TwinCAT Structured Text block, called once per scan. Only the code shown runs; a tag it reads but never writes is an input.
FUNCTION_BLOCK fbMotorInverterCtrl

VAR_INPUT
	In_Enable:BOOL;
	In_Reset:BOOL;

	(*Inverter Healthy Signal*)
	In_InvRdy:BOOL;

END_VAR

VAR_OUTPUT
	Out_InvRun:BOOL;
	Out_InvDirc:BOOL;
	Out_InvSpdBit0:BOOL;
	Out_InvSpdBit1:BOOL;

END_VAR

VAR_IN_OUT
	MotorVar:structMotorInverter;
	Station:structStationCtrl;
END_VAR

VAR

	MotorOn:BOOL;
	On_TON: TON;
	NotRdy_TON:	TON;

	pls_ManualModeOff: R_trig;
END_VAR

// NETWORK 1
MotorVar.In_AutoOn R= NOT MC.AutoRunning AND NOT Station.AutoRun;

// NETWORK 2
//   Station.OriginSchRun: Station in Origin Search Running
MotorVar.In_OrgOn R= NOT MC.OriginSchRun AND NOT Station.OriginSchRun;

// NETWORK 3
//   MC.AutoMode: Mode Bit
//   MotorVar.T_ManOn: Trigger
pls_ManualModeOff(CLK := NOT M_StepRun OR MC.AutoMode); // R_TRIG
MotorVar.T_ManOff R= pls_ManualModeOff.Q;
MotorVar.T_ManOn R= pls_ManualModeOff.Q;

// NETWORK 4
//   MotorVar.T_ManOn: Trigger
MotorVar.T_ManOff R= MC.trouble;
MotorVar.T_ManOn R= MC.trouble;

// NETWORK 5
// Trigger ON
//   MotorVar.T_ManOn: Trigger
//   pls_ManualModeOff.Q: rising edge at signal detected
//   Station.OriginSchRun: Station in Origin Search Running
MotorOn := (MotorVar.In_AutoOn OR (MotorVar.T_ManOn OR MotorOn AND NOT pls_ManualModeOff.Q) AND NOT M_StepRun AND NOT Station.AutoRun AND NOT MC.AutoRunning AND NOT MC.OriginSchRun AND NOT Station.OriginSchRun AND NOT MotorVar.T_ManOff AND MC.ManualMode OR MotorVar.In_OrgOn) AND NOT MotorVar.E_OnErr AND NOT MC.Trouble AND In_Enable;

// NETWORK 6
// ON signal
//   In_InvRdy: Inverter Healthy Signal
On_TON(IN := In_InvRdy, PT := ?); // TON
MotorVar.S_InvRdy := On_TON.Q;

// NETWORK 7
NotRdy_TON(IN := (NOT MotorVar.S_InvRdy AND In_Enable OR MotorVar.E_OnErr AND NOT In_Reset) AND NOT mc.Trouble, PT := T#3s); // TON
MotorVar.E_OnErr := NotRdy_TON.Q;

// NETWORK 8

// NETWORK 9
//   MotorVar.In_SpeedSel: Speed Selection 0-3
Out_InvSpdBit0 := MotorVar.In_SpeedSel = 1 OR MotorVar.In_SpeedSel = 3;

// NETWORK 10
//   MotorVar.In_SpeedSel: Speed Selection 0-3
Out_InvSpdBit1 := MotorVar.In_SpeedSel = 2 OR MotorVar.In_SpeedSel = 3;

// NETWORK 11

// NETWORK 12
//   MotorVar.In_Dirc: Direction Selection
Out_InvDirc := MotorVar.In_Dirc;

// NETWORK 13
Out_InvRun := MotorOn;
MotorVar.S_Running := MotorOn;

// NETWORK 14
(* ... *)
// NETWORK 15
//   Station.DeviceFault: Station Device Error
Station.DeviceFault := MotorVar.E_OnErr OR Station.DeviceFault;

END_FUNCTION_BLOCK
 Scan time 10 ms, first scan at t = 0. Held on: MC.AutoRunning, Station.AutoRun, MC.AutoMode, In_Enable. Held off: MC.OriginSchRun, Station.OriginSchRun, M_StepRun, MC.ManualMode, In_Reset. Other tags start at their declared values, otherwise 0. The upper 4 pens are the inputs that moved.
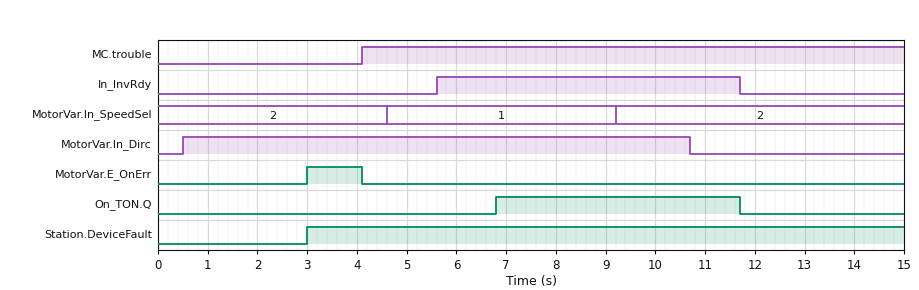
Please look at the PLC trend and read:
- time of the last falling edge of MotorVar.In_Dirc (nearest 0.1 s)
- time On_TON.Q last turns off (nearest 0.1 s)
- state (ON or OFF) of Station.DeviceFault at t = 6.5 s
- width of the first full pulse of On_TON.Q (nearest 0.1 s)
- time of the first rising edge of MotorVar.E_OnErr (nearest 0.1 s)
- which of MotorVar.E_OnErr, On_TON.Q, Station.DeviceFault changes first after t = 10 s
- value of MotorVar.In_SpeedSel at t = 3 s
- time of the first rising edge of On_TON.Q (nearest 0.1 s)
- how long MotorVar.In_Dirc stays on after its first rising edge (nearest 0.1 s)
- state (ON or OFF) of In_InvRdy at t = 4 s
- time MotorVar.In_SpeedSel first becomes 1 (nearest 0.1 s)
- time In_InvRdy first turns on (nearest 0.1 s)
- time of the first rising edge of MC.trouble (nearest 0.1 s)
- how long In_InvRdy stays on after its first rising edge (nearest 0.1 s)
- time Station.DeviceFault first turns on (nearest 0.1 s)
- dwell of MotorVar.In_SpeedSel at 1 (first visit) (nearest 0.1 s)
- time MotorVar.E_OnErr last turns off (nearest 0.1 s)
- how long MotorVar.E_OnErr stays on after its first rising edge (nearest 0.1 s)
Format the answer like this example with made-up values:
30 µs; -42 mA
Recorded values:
10.7 s; 11.7 s; ON; 4.9 s; 3.0 s; On_TON.Q; 2; 6.8 s; 10.2 s; OFF; 4.6 s; 5.6 s; 4.1 s; 6.1 s; 3.0 s; 4.6 s; 4.1 s; 1.1 s
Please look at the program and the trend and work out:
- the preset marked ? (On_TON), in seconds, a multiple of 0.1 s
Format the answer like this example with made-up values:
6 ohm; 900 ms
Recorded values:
1.2 s
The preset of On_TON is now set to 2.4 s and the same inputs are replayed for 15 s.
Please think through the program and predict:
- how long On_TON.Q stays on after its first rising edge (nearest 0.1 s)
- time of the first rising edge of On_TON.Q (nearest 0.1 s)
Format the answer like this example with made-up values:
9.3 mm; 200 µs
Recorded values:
3.7 s; 8.0 s
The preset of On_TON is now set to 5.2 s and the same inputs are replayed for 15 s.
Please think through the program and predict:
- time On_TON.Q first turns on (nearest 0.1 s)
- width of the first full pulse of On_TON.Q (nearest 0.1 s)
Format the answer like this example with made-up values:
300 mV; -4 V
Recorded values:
10.8 s; 0.9 s
